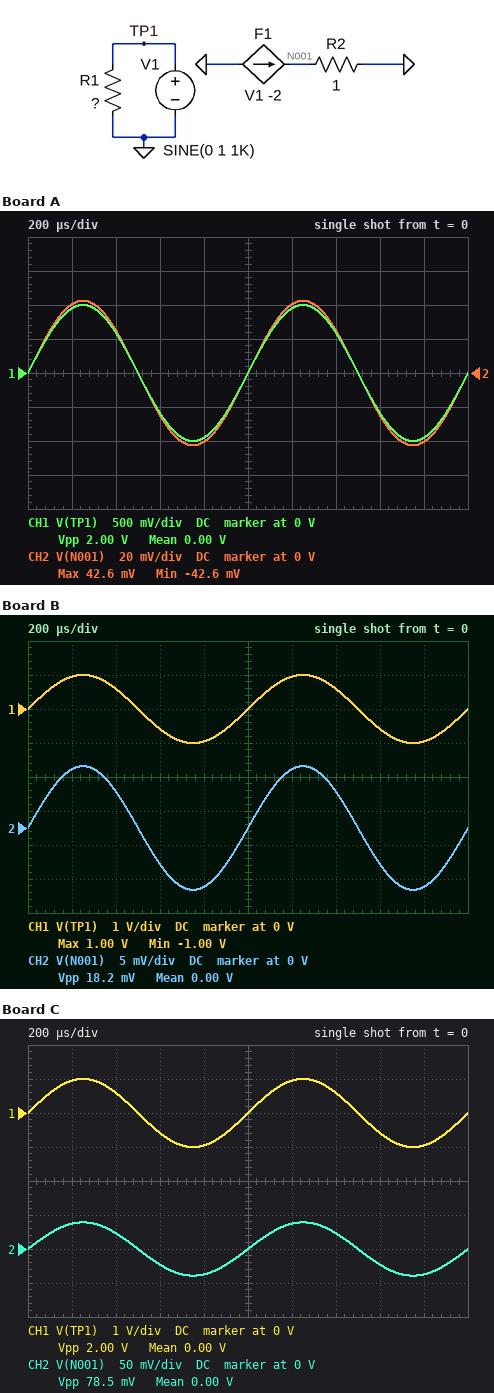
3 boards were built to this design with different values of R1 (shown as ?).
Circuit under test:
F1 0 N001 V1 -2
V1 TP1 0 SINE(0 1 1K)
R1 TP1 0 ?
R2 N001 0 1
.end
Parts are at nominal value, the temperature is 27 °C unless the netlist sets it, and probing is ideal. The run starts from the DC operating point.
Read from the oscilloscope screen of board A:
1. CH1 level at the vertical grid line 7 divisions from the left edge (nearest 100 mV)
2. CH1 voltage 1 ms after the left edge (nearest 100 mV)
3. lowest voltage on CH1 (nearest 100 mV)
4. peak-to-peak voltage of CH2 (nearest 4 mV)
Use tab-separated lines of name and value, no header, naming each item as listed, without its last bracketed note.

CH1 level at the vertical grid line 7 divisions from the left edge	600 mV
CH1 voltage 1 ms after the left edge	0 V
lowest voltage on CH1	-1.0 V
peak-to-peak voltage of CH2	84 mV
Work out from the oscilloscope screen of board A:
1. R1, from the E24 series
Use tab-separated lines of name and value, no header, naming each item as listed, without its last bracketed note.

R1, from the E24 series	47 Ω
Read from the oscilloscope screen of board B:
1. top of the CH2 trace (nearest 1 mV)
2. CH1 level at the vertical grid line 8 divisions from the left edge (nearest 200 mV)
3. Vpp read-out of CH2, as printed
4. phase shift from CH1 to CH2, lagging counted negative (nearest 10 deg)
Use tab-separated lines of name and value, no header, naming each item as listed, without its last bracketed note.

top of the CH2 trace	9 mV
CH1 level at the vertical grid line 8 divisions from the left edge	-600 mV
Vpp read-out of CH2, as printed	18.2 mV
phase shift from CH1 to CH2, lagging counted negative	0 deg
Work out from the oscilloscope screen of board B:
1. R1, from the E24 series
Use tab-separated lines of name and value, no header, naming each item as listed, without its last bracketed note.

R1, from the E24 series	220 Ω
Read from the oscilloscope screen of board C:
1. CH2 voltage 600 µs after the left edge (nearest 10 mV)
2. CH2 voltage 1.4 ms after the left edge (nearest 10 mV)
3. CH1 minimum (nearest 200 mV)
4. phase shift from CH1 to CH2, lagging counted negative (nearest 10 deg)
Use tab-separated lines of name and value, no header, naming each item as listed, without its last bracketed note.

CH2 voltage 600 µs after the left edge	-20 mV
CH2 voltage 1.4 ms after the left edge	20 mV
CH1 minimum	-1.0 V
phase shift from CH1 to CH2, lagging counted negative	0 deg
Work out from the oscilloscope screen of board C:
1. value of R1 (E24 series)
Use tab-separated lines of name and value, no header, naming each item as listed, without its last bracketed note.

value of R1	51 Ω
